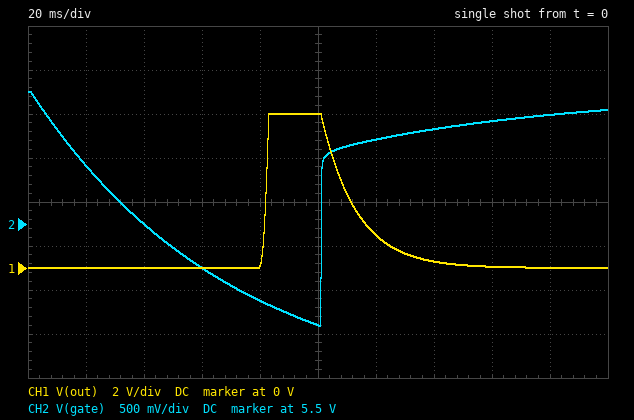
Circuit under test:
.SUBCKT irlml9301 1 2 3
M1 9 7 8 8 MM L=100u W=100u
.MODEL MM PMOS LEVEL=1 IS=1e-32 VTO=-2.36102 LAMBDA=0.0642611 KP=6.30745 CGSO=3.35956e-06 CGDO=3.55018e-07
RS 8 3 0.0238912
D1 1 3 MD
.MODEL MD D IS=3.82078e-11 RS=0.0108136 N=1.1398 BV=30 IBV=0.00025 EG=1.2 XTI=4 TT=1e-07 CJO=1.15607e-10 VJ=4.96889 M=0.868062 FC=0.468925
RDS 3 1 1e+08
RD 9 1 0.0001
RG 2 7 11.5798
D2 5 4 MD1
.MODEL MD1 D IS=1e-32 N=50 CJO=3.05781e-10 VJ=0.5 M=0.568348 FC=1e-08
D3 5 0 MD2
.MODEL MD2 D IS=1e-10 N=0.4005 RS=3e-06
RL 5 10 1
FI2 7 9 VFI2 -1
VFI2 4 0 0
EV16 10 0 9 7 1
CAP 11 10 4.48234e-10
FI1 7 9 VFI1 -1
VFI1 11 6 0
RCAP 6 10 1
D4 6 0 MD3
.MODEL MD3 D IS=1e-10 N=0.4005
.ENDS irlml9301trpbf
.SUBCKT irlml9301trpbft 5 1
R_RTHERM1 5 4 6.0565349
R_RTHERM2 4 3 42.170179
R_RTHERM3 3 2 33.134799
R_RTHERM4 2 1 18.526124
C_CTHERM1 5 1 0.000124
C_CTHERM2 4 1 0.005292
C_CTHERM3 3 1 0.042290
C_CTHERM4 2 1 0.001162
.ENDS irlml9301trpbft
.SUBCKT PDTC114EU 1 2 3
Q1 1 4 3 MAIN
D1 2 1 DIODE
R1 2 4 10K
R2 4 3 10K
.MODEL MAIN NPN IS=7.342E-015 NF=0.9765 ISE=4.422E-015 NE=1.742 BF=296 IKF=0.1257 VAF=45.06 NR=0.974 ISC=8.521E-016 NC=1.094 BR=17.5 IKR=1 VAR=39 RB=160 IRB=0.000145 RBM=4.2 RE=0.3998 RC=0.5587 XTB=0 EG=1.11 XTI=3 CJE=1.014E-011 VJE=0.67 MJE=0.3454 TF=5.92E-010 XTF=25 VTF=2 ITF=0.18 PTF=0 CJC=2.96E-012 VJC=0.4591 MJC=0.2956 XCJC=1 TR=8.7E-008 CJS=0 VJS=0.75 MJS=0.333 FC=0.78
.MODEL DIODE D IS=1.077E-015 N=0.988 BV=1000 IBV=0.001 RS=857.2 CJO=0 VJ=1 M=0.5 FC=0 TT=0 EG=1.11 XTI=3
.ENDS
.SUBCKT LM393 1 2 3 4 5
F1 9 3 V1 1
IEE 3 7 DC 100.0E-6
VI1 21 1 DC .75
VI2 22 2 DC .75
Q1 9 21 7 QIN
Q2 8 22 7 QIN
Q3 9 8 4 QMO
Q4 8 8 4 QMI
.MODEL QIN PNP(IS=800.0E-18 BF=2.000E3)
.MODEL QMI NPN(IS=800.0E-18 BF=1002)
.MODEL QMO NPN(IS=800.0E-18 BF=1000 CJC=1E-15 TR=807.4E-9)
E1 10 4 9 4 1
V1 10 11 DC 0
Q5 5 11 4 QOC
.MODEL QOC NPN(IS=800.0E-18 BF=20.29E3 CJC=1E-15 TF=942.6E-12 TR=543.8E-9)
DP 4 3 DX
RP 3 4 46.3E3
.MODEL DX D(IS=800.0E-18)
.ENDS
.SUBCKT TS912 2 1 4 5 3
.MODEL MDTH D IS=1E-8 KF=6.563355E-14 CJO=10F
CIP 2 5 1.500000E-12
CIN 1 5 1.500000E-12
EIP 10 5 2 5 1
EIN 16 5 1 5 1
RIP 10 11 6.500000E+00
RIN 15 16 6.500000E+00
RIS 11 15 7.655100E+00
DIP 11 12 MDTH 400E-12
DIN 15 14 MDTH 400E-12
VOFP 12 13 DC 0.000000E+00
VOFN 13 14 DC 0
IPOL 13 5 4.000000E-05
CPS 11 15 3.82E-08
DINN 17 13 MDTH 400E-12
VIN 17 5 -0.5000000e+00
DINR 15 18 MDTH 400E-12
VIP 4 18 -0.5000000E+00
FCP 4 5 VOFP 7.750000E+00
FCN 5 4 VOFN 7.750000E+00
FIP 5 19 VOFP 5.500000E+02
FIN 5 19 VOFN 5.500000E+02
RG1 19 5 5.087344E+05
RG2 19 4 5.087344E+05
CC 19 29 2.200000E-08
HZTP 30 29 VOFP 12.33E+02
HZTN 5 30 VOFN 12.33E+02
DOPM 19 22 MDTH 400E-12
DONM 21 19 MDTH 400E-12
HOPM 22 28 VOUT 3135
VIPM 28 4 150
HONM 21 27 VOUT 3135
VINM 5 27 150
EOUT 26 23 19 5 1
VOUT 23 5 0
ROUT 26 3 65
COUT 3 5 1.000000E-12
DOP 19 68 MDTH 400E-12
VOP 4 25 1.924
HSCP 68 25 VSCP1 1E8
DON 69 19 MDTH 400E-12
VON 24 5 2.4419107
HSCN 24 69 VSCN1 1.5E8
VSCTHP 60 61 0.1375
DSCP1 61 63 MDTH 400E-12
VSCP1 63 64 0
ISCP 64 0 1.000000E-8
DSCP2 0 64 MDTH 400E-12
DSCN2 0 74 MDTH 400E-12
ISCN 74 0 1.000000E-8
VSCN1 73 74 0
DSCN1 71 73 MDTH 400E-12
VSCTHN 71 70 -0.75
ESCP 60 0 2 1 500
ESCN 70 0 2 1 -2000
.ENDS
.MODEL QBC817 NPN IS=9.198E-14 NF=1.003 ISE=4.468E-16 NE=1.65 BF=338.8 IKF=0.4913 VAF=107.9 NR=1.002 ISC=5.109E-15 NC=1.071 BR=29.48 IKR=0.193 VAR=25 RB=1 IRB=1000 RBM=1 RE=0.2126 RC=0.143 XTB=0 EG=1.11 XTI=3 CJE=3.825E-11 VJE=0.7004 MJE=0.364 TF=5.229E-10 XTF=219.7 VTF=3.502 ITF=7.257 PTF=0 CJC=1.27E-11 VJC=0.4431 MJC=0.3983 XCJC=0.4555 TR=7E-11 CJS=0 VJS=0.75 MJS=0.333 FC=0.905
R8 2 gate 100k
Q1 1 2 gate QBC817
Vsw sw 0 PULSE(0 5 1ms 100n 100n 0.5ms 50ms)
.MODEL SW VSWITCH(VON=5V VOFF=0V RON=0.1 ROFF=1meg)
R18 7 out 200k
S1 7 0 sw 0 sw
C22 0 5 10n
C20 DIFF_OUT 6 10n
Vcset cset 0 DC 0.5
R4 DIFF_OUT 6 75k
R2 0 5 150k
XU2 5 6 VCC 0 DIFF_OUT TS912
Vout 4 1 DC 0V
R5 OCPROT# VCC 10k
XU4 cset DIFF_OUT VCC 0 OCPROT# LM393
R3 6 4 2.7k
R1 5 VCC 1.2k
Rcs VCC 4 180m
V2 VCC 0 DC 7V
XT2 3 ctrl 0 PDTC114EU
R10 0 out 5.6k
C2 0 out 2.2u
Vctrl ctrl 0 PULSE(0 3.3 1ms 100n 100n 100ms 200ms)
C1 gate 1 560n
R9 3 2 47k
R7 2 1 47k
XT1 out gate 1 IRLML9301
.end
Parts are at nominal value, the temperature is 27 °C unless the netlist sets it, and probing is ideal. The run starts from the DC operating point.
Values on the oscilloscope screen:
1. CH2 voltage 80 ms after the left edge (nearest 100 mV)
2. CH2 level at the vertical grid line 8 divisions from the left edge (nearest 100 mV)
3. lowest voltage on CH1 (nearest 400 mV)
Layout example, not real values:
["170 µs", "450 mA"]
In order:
["4.6 V", "6.7 V", "0 V"]
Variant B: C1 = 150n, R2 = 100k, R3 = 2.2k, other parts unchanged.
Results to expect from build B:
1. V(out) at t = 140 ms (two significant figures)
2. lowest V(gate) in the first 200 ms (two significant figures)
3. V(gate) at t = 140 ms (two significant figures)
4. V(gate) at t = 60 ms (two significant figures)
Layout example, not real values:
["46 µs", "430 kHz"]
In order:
["290 mV", "3.5 V", "6.9 V", "3.7 V"]
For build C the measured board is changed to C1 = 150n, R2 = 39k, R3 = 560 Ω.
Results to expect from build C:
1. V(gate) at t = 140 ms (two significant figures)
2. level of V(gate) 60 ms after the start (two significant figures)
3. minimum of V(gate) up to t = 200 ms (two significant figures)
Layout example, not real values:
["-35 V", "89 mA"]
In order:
["6.9 V", "3.7 V", "3.5 V"]
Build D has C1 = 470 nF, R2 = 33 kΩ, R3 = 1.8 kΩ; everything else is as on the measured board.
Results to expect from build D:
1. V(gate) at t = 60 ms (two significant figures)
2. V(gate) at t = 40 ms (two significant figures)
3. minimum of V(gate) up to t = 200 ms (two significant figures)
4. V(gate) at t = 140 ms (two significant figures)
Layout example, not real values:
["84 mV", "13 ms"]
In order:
["4.8 V", "5.3 V", "4.1 V", "6.6 V"]
